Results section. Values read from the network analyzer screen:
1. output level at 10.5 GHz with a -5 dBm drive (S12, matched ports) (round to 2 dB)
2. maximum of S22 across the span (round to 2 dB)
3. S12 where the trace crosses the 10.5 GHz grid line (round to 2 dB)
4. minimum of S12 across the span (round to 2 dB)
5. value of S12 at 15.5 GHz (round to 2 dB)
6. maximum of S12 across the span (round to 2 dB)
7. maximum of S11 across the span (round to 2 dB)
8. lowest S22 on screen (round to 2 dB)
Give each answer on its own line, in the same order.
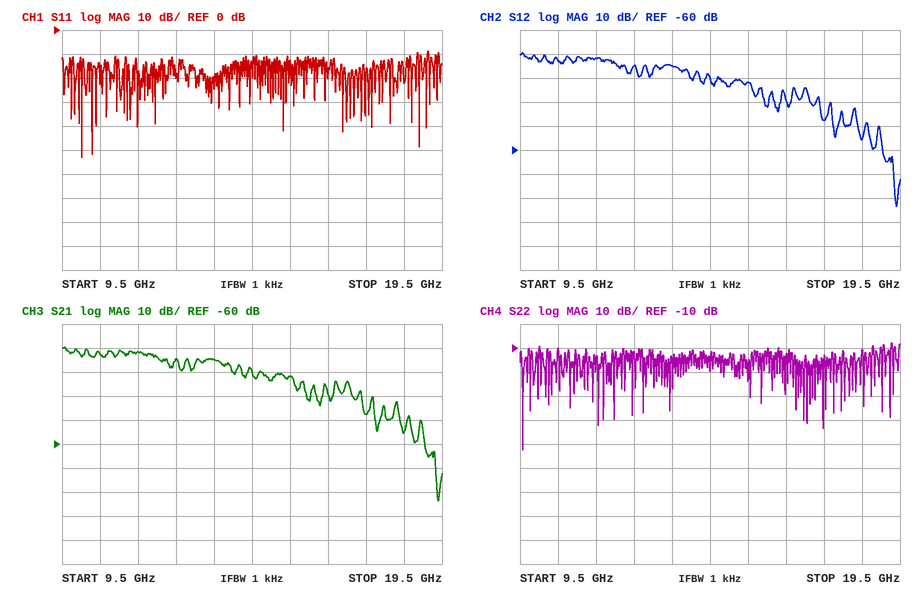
-28 dBm
-8 dB
-22 dB
-84 dB
-32 dB
-20 dB
-8 dB
-52 dB
